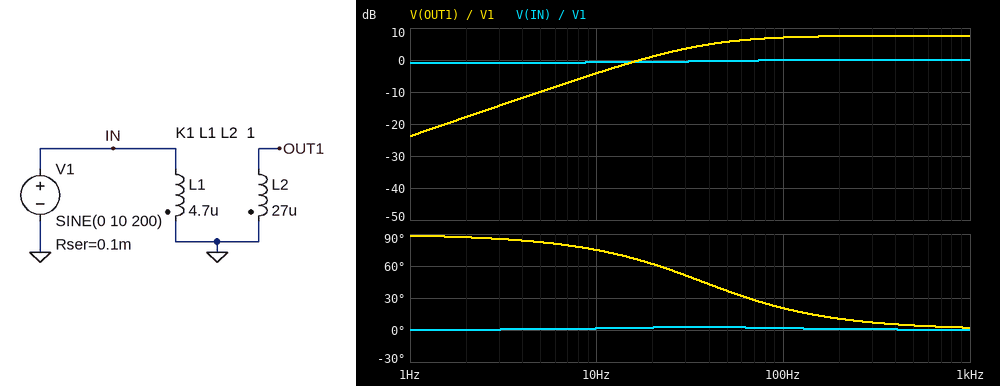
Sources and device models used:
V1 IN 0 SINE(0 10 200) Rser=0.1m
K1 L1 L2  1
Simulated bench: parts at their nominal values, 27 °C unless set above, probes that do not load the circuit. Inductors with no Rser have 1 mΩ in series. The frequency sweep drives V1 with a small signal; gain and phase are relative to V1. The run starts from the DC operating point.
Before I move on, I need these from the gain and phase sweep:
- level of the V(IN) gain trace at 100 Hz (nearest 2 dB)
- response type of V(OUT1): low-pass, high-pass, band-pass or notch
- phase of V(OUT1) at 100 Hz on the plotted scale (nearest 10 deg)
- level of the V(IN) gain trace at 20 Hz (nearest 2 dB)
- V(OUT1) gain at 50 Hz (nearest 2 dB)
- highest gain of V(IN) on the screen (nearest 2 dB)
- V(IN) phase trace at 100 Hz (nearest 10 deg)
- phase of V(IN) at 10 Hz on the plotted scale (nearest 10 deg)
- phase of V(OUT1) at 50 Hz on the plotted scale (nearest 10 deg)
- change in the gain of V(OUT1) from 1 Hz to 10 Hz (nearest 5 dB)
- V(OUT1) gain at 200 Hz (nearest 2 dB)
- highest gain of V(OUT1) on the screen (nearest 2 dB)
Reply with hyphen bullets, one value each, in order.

- 0 dB
- high-pass
- 20 deg
- 0 dB
- 6 dB
- 0 dB
- 0 deg
- 0 deg
- 40 deg
- 20 dB
- 8 dB
- 8 dB
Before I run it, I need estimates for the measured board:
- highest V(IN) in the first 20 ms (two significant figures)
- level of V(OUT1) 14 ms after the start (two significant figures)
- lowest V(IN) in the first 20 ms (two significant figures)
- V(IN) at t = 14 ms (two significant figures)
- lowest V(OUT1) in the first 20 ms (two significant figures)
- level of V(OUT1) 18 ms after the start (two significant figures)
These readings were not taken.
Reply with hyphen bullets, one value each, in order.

- 10 V
- -21 V
- -10 V
- -9.4 V
- -25 V
- -17 V
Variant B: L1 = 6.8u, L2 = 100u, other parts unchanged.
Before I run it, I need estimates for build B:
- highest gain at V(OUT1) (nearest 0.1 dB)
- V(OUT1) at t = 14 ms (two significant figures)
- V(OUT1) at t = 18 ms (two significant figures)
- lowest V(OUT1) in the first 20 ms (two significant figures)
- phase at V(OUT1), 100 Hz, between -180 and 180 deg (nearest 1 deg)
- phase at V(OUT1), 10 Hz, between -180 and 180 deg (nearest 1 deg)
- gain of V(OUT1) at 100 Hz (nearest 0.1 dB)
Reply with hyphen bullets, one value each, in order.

- 11.7 dB
- -35 V
- -26 V
- -41 V
- 14 deg
- 69 deg
- 11.4 dB
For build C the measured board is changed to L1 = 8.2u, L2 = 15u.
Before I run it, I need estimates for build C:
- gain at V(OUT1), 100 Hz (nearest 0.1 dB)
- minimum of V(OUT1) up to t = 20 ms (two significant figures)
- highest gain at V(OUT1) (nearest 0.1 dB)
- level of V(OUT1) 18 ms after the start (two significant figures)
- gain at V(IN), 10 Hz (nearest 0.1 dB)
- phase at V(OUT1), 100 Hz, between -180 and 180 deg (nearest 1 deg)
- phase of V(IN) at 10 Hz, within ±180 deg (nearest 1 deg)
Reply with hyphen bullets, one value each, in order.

- 2.4 dB
- -14 V
- 2.6 dB
- -9.1 V
- -0.7 dB
- 12 deg
- 2 deg
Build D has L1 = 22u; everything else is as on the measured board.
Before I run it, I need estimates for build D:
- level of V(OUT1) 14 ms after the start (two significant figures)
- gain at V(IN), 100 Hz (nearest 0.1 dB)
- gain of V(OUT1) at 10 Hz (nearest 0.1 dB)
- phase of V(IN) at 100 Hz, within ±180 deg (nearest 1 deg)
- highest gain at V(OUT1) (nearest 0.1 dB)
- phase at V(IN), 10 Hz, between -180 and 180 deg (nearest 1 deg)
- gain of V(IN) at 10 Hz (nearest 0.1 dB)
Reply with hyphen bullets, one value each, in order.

- -11 V
- 0 dB
- -1.2 dB
- 0 deg
- 0.9 dB
- 3 deg
- -0.3 dB
